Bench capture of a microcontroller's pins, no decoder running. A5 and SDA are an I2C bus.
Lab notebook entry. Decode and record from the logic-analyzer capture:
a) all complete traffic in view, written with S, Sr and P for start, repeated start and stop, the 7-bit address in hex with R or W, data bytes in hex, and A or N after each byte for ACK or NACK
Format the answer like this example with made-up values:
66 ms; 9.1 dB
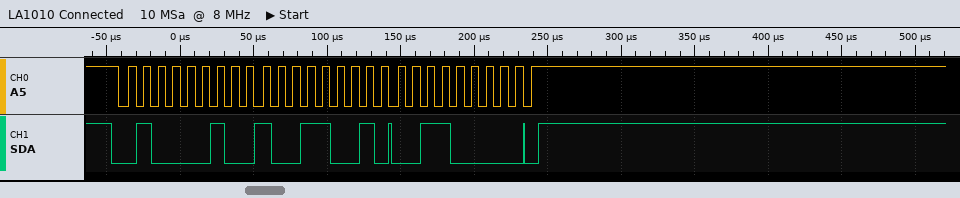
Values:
S 21W A 99 A 30 A P
